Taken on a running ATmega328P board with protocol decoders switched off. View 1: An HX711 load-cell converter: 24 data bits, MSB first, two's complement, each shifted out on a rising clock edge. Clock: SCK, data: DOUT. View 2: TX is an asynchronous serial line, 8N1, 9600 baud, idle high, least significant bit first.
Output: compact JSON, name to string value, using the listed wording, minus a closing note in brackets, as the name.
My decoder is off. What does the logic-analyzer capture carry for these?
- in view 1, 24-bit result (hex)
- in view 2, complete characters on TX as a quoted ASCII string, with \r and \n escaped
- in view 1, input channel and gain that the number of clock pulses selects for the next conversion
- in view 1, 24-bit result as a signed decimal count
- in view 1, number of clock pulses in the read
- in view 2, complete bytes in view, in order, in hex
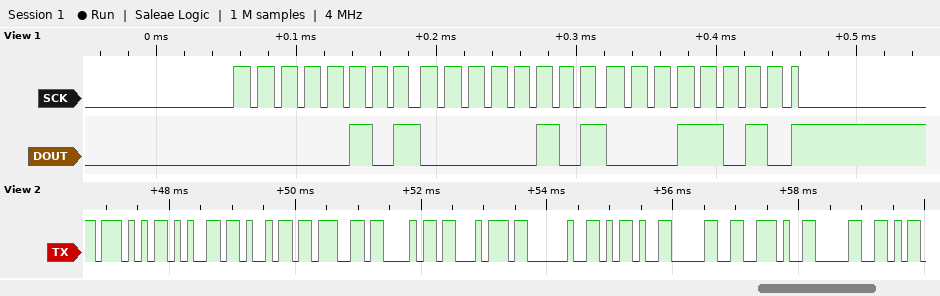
{"in view 1, 24-bit result": "0x05051A", "in view 2, complete characters on TX as a quoted ASCII string, with \\r and \\n escaped": "\"Weight -0.0\"", "in view 1, input channel and gain that the number of clock pulses selects for the next conversion": "channel A, gain 128", "in view 1, 24-bit result as a signed decimal count": "328986", "in view 1, number of clock pulses in the read": "25", "in view 2, complete bytes in view, in order, in hex": "57 65 69 67 68 74 20 2D 30 2E 30"}
